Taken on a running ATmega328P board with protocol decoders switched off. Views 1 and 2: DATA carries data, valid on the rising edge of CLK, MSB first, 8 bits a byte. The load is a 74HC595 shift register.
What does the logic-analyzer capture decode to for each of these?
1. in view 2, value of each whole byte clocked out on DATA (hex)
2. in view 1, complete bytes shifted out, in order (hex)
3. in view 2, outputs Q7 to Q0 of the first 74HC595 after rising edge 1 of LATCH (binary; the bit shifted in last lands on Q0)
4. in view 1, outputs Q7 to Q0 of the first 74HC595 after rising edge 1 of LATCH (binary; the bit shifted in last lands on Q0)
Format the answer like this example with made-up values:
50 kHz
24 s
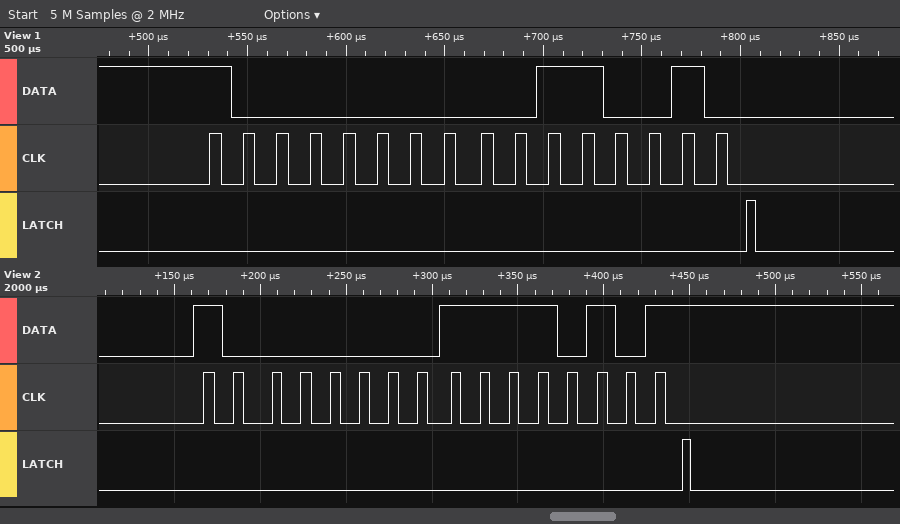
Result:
80 F5
80 32
11110101
00110010
